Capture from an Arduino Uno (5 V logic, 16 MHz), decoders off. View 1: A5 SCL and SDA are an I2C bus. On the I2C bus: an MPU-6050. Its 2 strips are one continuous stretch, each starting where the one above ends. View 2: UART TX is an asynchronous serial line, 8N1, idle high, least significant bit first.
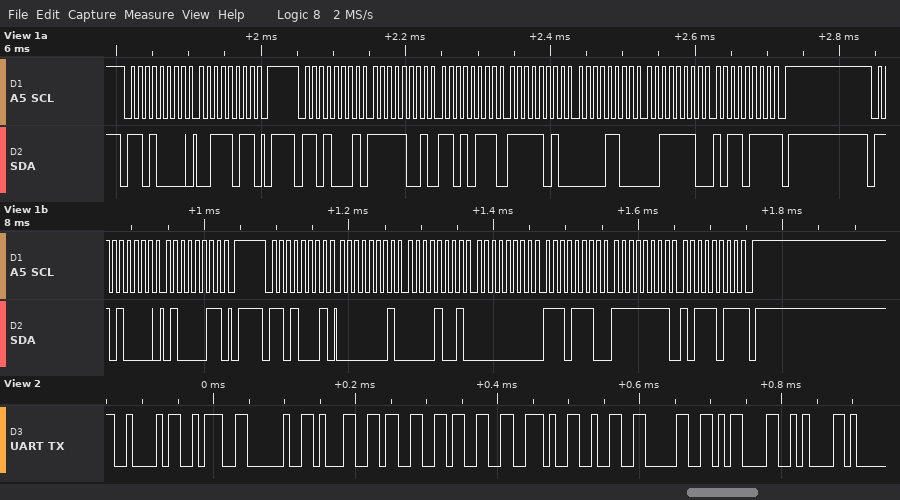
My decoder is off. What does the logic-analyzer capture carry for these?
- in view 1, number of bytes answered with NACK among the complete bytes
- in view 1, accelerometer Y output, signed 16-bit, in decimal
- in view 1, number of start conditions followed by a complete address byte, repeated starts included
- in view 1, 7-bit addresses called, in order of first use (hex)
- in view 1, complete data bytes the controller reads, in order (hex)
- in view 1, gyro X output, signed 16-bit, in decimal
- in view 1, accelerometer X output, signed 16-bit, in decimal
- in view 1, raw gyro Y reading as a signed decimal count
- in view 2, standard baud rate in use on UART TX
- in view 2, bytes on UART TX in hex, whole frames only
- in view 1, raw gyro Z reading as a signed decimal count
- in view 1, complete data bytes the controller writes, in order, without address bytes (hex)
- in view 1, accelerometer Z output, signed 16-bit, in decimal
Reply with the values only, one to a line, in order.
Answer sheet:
2
-1524
4
0x68
F9 D7 FA 0C 3E B7 01 09 00 EE FF BB
265
-1577
238
115200 baud
42 3A 20 31 33 33 2E 32 30 0D 0A
-69
3B 43
16055
